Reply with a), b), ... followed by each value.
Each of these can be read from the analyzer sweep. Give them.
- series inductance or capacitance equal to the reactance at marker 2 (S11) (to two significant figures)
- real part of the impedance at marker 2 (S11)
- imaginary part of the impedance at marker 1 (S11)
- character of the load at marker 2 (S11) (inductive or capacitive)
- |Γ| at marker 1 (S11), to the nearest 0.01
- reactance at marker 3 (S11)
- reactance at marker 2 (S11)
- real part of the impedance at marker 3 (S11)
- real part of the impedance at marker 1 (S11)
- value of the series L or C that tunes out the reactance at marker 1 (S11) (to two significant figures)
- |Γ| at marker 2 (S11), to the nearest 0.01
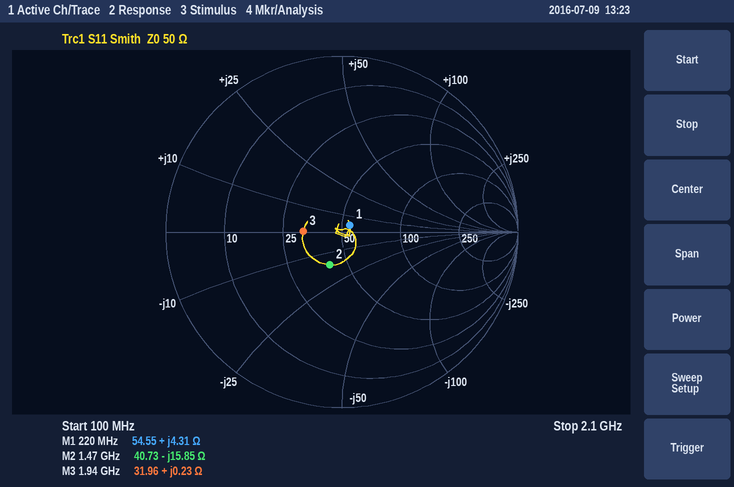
a) 6.8 pF
b) 40.73 Ω
c) +4.31 Ω
d) capacitive
e) 0.06
f) +0.23 Ω
g) -15.85 Ω
h) 31.96 Ω
i) 54.55 Ω
j) 170 pF
k) 0.20
